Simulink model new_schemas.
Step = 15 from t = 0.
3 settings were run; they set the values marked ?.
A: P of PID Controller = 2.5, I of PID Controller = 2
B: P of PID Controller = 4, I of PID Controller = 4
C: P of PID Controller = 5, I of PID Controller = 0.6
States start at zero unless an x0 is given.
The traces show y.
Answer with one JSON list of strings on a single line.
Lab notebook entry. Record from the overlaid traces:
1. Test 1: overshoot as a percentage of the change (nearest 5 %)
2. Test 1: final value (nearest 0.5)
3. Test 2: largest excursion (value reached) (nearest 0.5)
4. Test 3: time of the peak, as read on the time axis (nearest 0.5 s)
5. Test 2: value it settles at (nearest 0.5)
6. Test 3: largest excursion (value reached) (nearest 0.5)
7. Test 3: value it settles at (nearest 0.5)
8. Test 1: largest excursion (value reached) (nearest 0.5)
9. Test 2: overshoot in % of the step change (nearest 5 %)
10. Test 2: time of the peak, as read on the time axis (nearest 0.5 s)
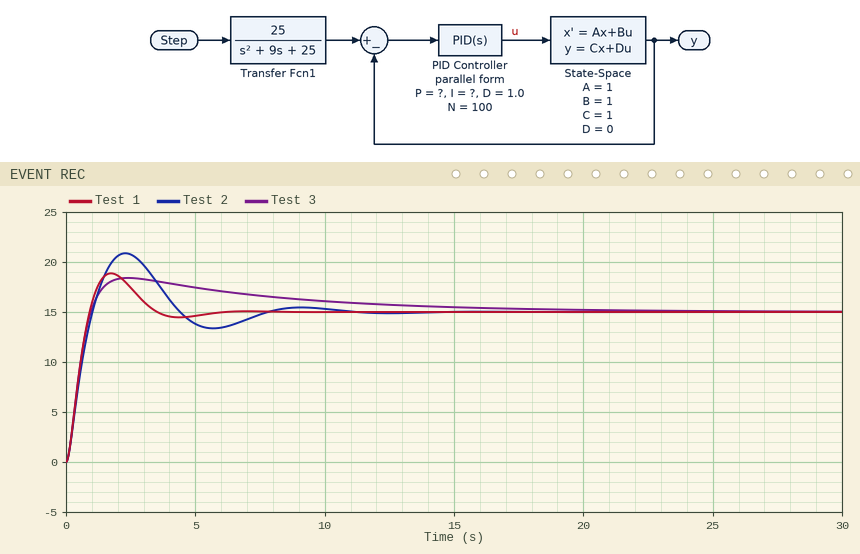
["25 %", "15.0", "21.0", "2.5 s", "15.0", "18.5", "15.0", "19.0", "40 %", "2.5 s"]
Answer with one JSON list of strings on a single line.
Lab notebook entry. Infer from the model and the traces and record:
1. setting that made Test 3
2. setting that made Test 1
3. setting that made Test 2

["C", "B", "A"]
